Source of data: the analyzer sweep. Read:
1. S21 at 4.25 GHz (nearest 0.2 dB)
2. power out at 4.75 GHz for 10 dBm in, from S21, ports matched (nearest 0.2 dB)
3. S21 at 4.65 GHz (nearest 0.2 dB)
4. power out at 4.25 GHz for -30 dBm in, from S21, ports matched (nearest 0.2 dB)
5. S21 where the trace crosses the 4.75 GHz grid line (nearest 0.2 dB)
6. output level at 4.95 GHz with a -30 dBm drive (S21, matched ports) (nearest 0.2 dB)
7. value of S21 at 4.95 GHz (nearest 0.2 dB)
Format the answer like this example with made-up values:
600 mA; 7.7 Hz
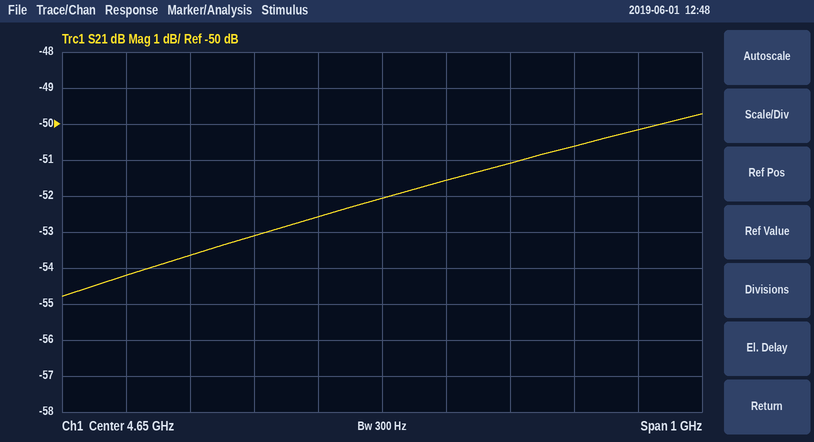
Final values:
-54.2 dB; -41.6 dBm; -52.0 dB; -84.2 dBm; -51.6 dB; -80.6 dBm; -50.6 dB
